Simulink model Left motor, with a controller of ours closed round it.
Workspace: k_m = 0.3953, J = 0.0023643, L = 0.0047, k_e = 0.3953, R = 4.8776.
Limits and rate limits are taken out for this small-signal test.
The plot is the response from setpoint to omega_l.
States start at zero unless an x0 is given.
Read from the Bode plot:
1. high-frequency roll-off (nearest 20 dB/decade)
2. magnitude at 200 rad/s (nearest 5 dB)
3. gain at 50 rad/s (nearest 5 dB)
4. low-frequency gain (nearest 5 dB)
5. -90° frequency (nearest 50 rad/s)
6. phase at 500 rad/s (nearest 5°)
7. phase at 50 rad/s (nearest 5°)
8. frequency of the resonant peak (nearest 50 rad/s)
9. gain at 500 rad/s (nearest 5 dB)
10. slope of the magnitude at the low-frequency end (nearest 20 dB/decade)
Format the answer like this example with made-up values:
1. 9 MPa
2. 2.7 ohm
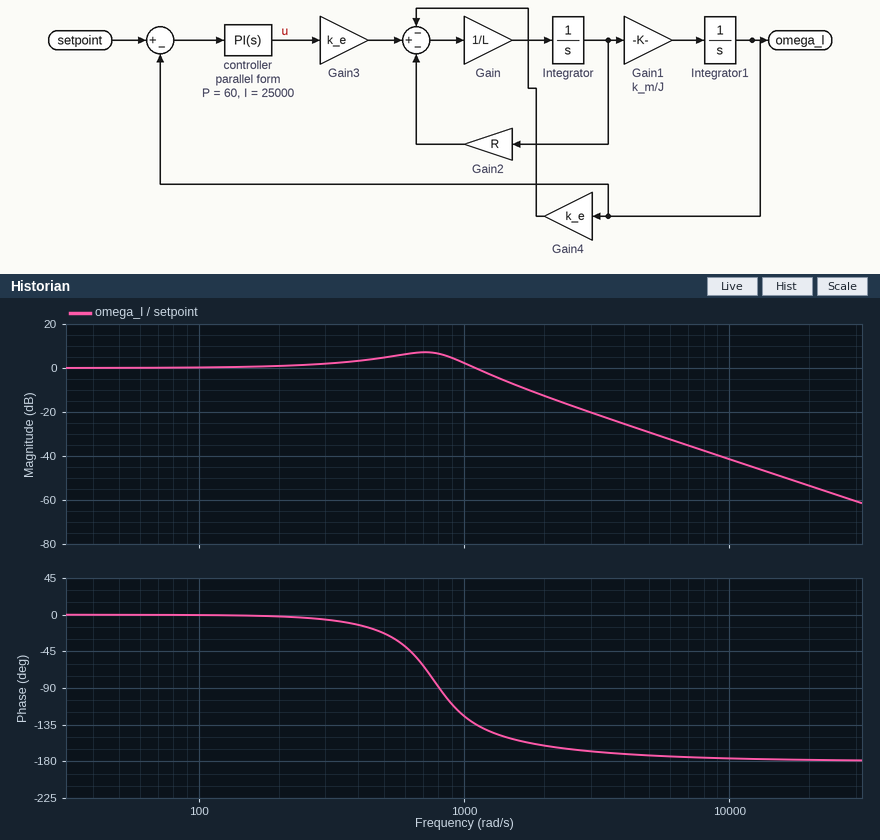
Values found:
1. -40 dB/decade
2. 0 dB
3. 0 dB
4. 0 dB
5. 800 rad/s
6. -25°
7. 0°
8. 700 rad/s
9. 5 dB
10. 0 dB/decade
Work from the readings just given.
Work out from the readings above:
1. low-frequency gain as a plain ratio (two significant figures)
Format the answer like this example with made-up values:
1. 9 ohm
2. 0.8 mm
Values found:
1. 1.0
